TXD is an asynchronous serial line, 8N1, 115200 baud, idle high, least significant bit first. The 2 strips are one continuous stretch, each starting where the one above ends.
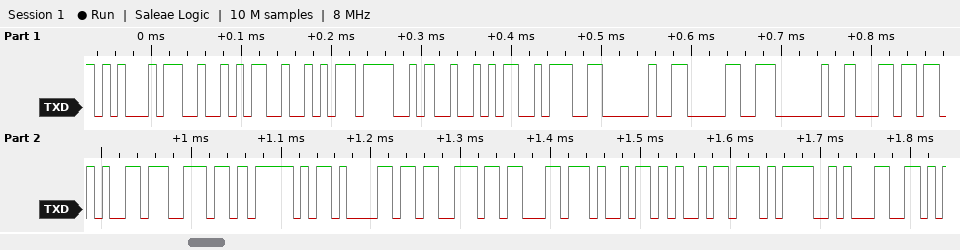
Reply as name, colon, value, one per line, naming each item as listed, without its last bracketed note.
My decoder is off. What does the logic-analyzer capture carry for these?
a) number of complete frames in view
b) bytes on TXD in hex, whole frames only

number of complete frames in view: 20
bytes on TXD in hex, whole frames only: 45 52 52 4F 52 3A 20 30 20 6C 65 6E 5F 61 73 63 69 69 3D 31
